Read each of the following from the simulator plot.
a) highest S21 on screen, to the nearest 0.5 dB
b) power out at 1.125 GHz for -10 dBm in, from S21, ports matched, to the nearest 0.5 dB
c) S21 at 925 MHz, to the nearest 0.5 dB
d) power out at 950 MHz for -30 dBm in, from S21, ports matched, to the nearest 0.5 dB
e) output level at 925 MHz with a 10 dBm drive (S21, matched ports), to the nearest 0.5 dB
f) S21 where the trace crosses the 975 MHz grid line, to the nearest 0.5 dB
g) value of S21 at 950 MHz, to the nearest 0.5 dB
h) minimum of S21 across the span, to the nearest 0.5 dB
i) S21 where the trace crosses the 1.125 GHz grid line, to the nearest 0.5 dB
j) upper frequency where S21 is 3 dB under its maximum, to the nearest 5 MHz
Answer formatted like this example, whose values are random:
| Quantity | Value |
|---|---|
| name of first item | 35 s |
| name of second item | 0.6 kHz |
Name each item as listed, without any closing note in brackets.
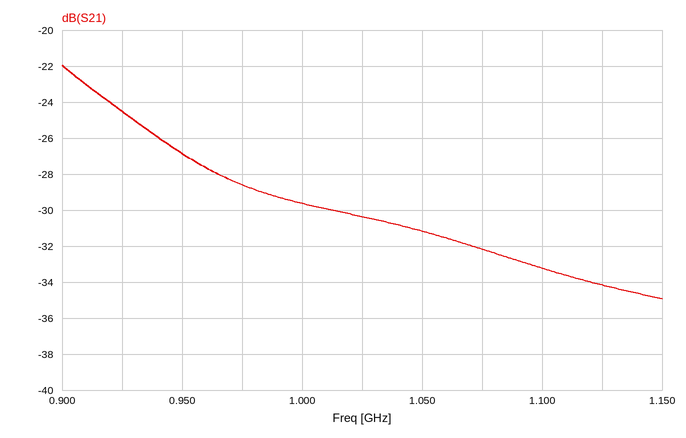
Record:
| Quantity | Value |
|---|---|
| highest S21 on screen, to the nearest 0.5 dB | -22.0 dB |
| power out at 1.125 GHz for -10 dBm in, from S21, ports matched, to the nearest 0.5 dB | -44.0 dBm |
| S21 at 925 MHz, to the nearest 0.5 dB | -24.5 dB |
| power out at 950 MHz for -30 dBm in, from S21, ports matched, to the nearest 0.5 dB | -57.0 dBm |
| output level at 925 MHz with a 10 dBm drive (S21, matched ports), to the nearest 0.5 dB | -14.5 dBm |
| S21 where the trace crosses the 975 MHz grid line, to the nearest 0.5 dB | -28.5 dB |
| value of S21 at 950 MHz, to the nearest 0.5 dB | -27.0 dB |
| minimum of S21 across the span, to the nearest 0.5 dB | -35.0 dB |
| S21 where the trace crosses the 1.125 GHz grid line, to the nearest 0.5 dB | -34.0 dB |
| upper frequency where S21 is 3 dB under its maximum, to the nearest 5 MHz | 930 MHz |
